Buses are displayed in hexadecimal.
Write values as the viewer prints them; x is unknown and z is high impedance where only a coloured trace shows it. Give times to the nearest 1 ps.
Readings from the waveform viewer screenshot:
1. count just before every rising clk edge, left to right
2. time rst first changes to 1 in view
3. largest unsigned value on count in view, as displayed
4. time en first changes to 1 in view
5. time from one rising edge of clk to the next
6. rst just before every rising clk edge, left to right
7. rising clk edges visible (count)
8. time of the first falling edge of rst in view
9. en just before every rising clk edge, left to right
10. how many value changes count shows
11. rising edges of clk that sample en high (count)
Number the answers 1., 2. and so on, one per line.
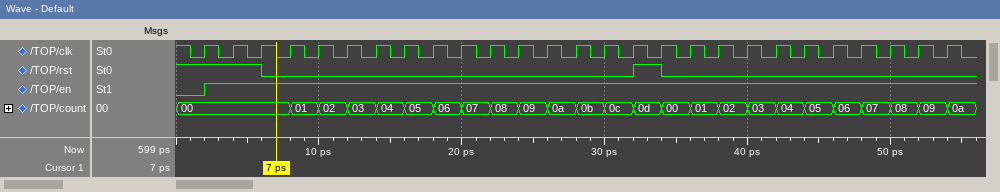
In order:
1. 00, 00, 00, 00, 01, 02, 03, 04, 05, 06, 07, 08, 09, 0a, 0b, 0c, 0d, 00, 01, 02, 03, 04, 05, 06, 07, 08, 09
2. 32 ps
3. 0d
4. 2 ps
5. 2 ps
6. 1 1 1 0 0 0 0 0 0 0 0 0 0 0 0 0 1 0 0 0 0 0 0 0 0 0 0
7. 27
8. 6 ps
9. 0 1 1 1 1 1 1 1 1 1 1 1 1 1 1 1 1 1 1 1 1 1 1 1 1 1 1
10. 24
11. 26
